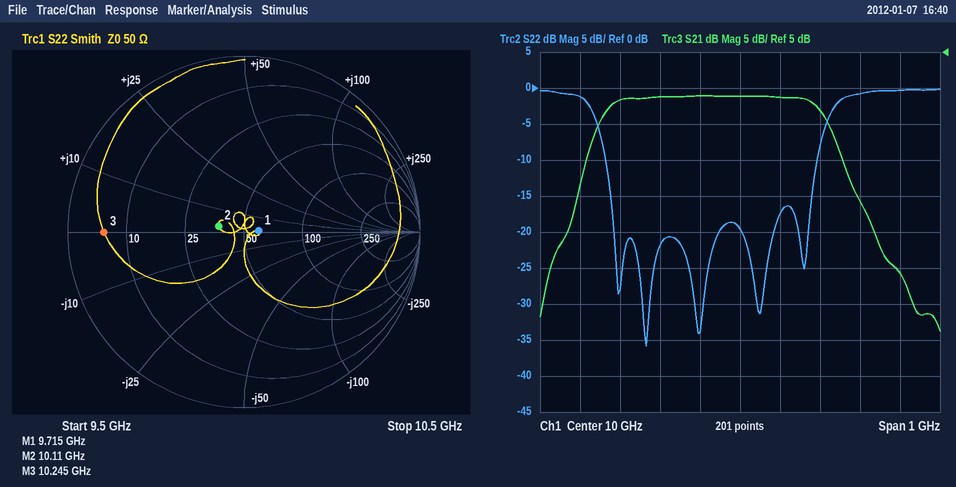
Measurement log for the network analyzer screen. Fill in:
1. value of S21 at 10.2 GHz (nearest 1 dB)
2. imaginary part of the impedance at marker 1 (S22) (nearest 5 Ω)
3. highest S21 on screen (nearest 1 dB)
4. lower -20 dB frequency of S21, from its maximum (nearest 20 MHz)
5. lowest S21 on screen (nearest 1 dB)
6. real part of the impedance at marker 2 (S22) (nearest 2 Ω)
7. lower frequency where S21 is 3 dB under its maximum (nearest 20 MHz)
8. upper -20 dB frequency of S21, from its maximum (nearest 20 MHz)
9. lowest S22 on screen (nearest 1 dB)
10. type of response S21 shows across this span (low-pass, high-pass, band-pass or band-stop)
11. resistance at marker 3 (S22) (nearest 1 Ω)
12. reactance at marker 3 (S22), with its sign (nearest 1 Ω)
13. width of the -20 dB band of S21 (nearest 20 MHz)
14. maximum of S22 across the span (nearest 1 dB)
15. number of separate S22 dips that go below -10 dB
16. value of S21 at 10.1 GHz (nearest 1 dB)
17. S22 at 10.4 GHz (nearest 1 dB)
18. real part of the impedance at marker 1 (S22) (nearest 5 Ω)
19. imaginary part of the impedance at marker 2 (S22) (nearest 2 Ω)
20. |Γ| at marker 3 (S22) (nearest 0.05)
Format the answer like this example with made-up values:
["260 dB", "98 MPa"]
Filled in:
["-3 dB", "0 Ω", "-1 dB", "9.56 GHz", "-34 dB", "38 Ω", "9.66 GHz", "10.34 GHz", "-36 dB", "band-pass", "6 Ω", "0 Ω", "780 MHz", "0 dB", "5", "-1 dB", "0 dB", "60 Ω", "+2 Ω", "0.80"]
